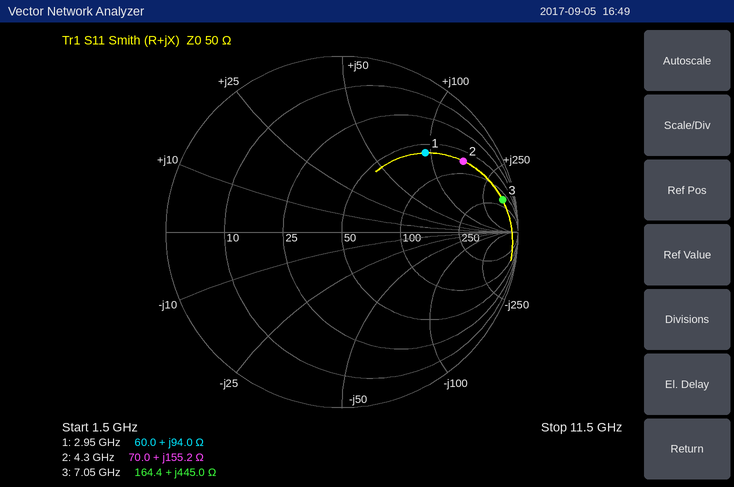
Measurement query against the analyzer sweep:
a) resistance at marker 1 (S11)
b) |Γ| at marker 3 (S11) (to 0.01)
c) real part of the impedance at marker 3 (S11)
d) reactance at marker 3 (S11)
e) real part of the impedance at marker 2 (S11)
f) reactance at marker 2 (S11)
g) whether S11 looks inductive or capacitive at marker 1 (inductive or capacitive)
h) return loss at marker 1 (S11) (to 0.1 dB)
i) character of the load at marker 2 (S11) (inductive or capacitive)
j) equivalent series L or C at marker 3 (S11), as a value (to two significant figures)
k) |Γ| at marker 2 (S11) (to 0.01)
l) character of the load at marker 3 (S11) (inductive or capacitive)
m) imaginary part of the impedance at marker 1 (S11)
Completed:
60.0 Ω
0.93
164.4 Ω
+445.0 Ω
70.0 Ω
+155.2 Ω
inductive
3.7 dB
inductive
10 nH
0.80
inductive
+94.0 Ω
